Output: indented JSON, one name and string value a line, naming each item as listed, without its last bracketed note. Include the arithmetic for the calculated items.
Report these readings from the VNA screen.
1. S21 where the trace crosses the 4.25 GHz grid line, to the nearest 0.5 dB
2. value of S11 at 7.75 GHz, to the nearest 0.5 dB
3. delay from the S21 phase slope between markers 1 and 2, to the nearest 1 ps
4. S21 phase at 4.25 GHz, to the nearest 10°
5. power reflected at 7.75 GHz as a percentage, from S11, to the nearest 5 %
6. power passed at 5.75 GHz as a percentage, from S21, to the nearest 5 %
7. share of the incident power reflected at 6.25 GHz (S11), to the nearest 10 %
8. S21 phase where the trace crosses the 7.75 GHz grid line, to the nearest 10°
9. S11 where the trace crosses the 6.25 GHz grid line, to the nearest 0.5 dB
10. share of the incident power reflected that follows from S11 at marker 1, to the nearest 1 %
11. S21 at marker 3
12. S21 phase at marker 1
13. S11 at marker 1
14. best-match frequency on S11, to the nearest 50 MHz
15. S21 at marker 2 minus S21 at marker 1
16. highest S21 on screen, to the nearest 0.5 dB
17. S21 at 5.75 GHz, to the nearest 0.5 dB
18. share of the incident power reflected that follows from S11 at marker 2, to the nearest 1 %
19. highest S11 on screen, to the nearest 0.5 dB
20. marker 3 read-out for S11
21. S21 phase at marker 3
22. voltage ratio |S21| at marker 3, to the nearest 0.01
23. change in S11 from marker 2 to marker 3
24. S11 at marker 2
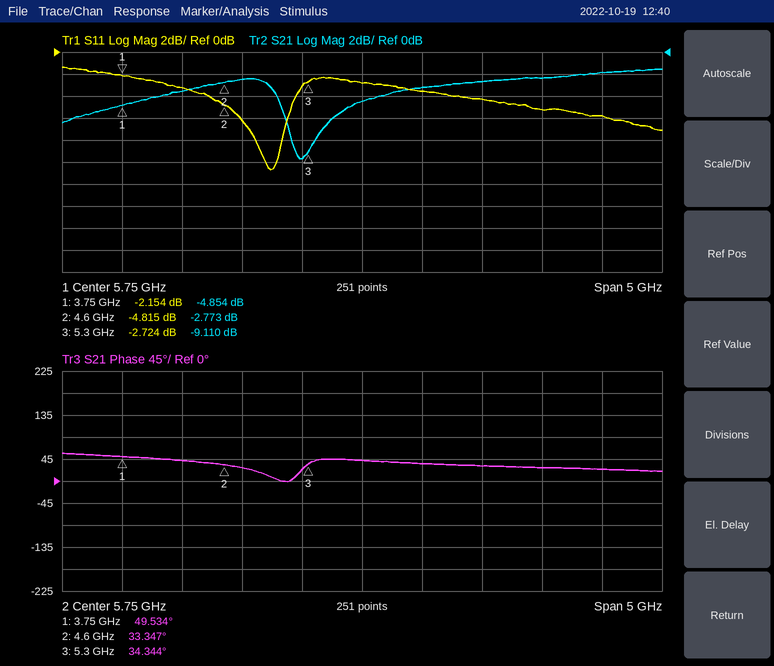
{
  "S21 where the trace crosses the 4.25 GHz grid line, to the nearest 0.5 dB": "-3.5 dB",
  "value of S11 at 7.75 GHz, to the nearest 0.5 dB": "-6.0 dB",
  "delay from the S21 phase slope between markers 1 and 2, to the nearest 1 ps": "−(33.347° − (49.534°))/(360° × 850 MHz) ≈ 53 ps",
  "S21 phase at 4.25 GHz, to the nearest 10°": "40°",
  "power reflected at 7.75 GHz as a percentage, from S11, to the nearest 5 %": "10^(-6/10) ≈ 25 %",
  "power passed at 5.75 GHz as a percentage, from S21, to the nearest 5 %": "10^(-4.5/10) ≈ 35 %",
  "share of the incident power reflected at 6.25 GHz (S11), to the nearest 10 %": "10^(-3.5/10) ≈ 44.7 %, so 40 % to the nearest 10 %",
  "S21 phase where the trace crosses the 7.75 GHz grid line, to the nearest 10°": "20°",
  "S11 where the trace crosses the 6.25 GHz grid line, to the nearest 0.5 dB": "-3.5 dB",
  "share of the incident power reflected that follows from S11 at marker 1, to the nearest 1 %": "10^(-2.154/10) ≈ 61 %",
  "S21 at marker 3": "-9.110 dB",
  "S21 phase at marker 1": "49.534°",
  "S11 at marker 1": "-2.154 dB",
  "best-match frequency on S11, to the nearest 50 MHz": "5.00 GHz",
  "S21 at marker 2 minus S21 at marker 1": "-2.773 − (-4.854) = 2.081 dB",
  "highest S21 on screen, to the nearest 0.5 dB": "-1.5 dB",
  "S21 at 5.75 GHz, to the nearest 0.5 dB": "-4.5 dB",
  "share of the incident power reflected that follows from S11 at marker 2, to the nearest 1 %": "10^(-4.815/10) ≈ 33 %",
  "highest S11 on screen, to the nearest 0.5 dB": "-1.5 dB",
  "marker 3 read-out for S11": "-2.724 dB",
  "S21 phase at marker 3": "34.344°",
  "voltage ratio |S21| at marker 3, to the nearest 0.01": "10^(-9.11/20) ≈ 0.35",
  "change in S11 from marker 2 to marker 3": "-2.724 − (-4.815) = 2.091 dB",
  "S11 at marker 2": "-4.815 dB"
}
